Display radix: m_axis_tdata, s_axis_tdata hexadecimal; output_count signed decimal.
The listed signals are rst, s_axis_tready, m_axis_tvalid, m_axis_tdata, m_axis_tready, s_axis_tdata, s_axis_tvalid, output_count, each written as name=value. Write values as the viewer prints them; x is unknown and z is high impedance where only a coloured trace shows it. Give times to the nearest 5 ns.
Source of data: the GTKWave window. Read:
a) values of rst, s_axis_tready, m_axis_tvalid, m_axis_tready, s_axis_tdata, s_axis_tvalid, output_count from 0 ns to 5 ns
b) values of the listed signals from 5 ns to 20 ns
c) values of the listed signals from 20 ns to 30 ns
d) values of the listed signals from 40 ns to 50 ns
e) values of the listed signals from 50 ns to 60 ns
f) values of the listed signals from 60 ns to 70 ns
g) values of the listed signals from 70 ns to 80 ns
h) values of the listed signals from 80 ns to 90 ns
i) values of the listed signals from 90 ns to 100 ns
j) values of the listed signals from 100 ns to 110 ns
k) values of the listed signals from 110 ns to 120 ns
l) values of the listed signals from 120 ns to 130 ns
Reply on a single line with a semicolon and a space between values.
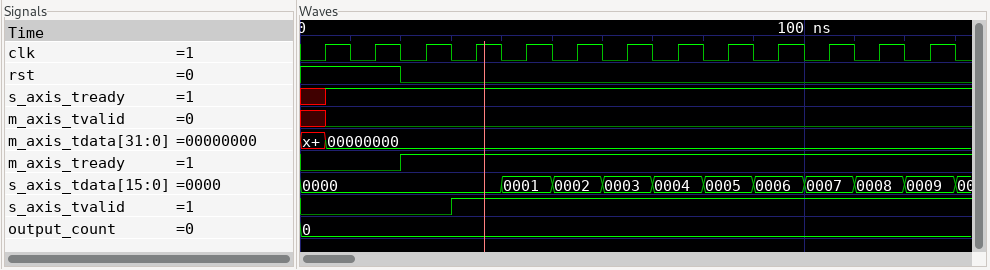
rst=1, s_axis_tready=x, m_axis_tvalid=x, m_axis_tready=0, s_axis_tdata=0000, s_axis_tvalid=0, output_count=0; rst=1, s_axis_tready=1, m_axis_tvalid=0, m_axis_tdata=00000000, m_axis_tready=0, s_axis_tdata=0000, s_axis_tvalid=0, output_count=0; rst=0, s_axis_tready=1, m_axis_tvalid=0, m_axis_tdata=00000000, m_axis_tready=1, s_axis_tdata=0000, s_axis_tvalid=0, output_count=0; rst=0, s_axis_tready=1, m_axis_tvalid=0, m_axis_tdata=00000000, m_axis_tready=1, s_axis_tdata=0001, s_axis_tvalid=1, output_count=0; rst=0, s_axis_tready=1, m_axis_tvalid=0, m_axis_tdata=00000000, m_axis_tready=1, s_axis_tdata=0002, s_axis_tvalid=1, output_count=0; rst=0, s_axis_tready=1, m_axis_tvalid=0, m_axis_tdata=00000000, m_axis_tready=1, s_axis_tdata=0003, s_axis_tvalid=1, output_count=0; rst=0, s_axis_tready=1, m_axis_tvalid=0, m_axis_tdata=00000000, m_axis_tready=1, s_axis_tdata=0004, s_axis_tvalid=1, output_count=0; rst=0, s_axis_tready=1, m_axis_tvalid=0, m_axis_tdata=00000000, m_axis_tready=1, s_axis_tdata=0005, s_axis_tvalid=1, output_count=0; rst=0, s_axis_tready=1, m_axis_tvalid=0, m_axis_tdata=00000000, m_axis_tready=1, s_axis_tdata=0006, s_axis_tvalid=1, output_count=0; rst=0, s_axis_tready=1, m_axis_tvalid=0, m_axis_tdata=00000000, m_axis_tready=1, s_axis_tdata=0007, s_axis_tvalid=1, output_count=0; rst=0, s_axis_tready=1, m_axis_tvalid=0, m_axis_tdata=00000000, m_axis_tready=1, s_axis_tdata=0008, s_axis_tvalid=1, output_count=0; rst=0, s_axis_tready=1, m_axis_tvalid=0, m_axis_tdata=00000000, m_axis_tready=1, s_axis_tdata=0009, s_axis_tvalid=1, output_count=0
